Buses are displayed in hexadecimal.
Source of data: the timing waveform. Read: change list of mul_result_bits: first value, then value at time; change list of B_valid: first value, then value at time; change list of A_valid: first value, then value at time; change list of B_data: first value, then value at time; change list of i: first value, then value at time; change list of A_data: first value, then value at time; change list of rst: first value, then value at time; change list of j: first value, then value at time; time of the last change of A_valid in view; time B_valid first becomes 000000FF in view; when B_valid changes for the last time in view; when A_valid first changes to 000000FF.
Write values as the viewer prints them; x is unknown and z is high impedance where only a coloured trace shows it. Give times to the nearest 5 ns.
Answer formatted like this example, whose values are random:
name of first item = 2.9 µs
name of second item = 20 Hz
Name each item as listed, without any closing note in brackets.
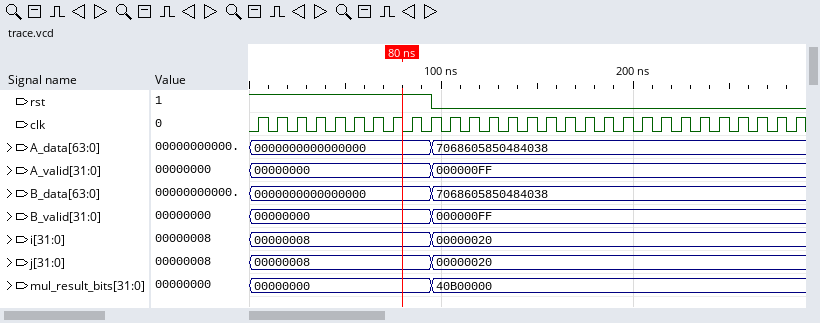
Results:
change list of mul_result_bits: first value, then value at time = 00000000, 40B00000 at 95 ns
change list of B_valid: first value, then value at time = 00000000, 000000FF at 95 ns
change list of A_valid: first value, then value at time = 00000000, 000000FF at 95 ns
change list of B_data: first value, then value at time = 0000000000000000, 7068605850484038 at 95 ns
change list of i: first value, then value at time = 00000008, 00000020 at 95 ns
change list of A_data: first value, then value at time = 0000000000000000, 7068605850484038 at 95 ns
change list of rst: first value, then value at time = 1, 0 at 95 ns
change list of j: first value, then value at time = 00000008, 00000020 at 95 ns
time of the last change of A_valid in view = 95 ns
time B_valid first becomes 000000FF in view = 95 ns
when B_valid changes for the last time in view = 95 ns
when A_valid first changes to 000000FF = 95 ns
